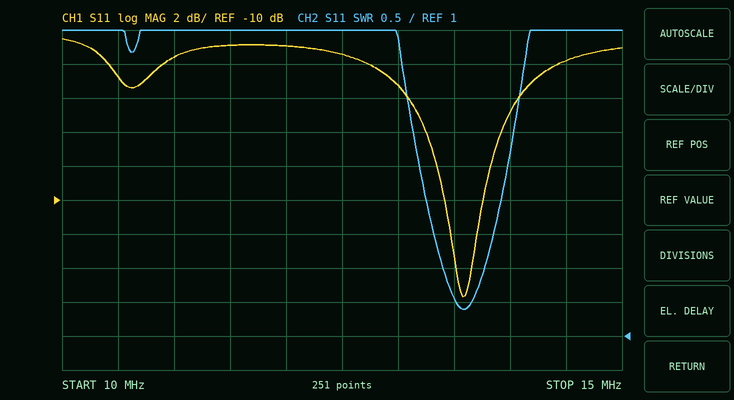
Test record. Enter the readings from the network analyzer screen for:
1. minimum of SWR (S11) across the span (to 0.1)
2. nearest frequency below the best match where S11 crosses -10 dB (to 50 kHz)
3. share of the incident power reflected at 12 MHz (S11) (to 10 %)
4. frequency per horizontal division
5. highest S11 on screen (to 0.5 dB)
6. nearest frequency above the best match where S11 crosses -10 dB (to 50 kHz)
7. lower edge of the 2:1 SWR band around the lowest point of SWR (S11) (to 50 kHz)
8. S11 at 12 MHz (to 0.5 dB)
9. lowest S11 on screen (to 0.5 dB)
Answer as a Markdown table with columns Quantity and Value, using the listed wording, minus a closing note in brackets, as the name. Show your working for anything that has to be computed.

| Quantity | Value |
|---|---|
| minimum of SWR (S11) across the span | 1.4 |
| nearest frequency below the best match where S11 crosses -10 dB | 13.40 MHz |
| share of the incident power reflected at 12 MHz (S11) | 10^(-1/10) ≈ 79.4 %, so 80 % to the nearest 10 % |
| frequency per horizontal division | 500 kHz |
| highest S11 on screen | -0.5 dB |
| nearest frequency above the best match where S11 crosses -10 dB | 13.75 MHz |
| lower edge of the 2:1 SWR band around the lowest point of SWR (S11) | 13.40 MHz |
| S11 at 12 MHz | -1.0 dB |
| lowest S11 on screen | -15.5 dB |
